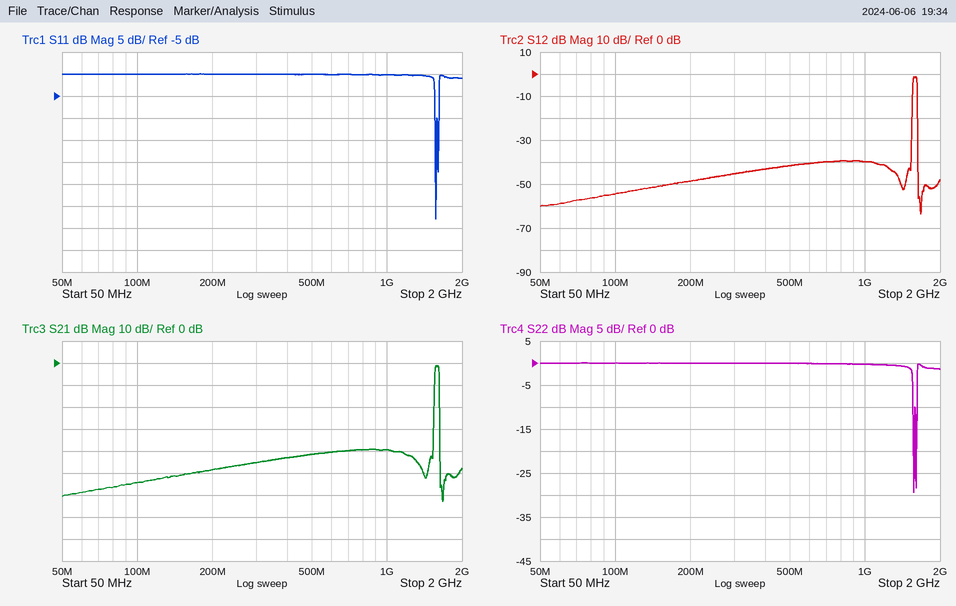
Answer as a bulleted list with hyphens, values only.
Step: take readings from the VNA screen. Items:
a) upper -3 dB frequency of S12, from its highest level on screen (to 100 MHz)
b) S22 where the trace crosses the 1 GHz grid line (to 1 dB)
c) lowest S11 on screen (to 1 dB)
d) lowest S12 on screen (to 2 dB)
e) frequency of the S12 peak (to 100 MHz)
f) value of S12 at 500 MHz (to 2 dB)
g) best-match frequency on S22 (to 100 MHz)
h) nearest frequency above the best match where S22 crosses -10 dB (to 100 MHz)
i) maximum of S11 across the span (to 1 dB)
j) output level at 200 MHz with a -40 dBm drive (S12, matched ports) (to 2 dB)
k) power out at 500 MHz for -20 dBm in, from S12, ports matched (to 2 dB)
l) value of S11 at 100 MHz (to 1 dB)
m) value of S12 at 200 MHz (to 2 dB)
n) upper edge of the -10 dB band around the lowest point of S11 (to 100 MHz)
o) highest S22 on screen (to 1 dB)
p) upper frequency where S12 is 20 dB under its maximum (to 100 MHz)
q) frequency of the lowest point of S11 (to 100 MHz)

- 1.6 GHz
- 0 dB
- -33 dB
- -64 dB
- 1.6 GHz
- -42 dB
- 1.6 GHz
- 1.6 GHz
- 0 dB
- -88 dBm
- -62 dBm
- 0 dB
- -48 dB
- 1.6 GHz
- 0 dB
- 1.6 GHz
- 1.6 GHz
